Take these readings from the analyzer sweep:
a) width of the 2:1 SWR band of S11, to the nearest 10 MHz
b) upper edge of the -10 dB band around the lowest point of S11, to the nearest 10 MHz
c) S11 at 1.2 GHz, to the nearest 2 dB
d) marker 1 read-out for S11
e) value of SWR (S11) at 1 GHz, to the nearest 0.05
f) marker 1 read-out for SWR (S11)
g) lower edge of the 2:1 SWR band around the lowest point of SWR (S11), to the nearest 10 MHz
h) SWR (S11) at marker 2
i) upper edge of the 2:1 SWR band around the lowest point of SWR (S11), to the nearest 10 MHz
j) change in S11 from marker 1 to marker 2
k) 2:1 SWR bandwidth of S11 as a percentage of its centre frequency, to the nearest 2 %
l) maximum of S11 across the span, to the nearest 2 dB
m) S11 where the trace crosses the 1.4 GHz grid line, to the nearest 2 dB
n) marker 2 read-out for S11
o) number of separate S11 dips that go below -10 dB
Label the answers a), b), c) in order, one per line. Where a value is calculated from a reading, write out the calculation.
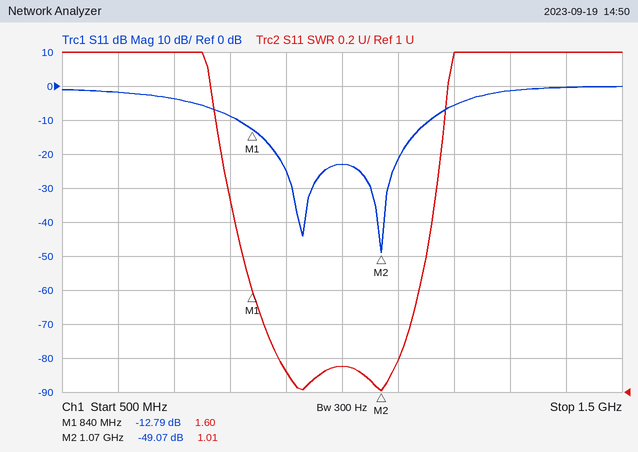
a) 1.16 GHz − 810 MHz = 350 MHz
b) 1.16 GHz
c) -6 dB
d) -12.79 dB
e) 1.15
f) 1.60
g) 810 MHz
h) 1.01
i) 1.16 GHz
j) -49.07 − (-12.79) = -36.28 dB
k) 350 MHz / 985 MHz ≈ 36 %
l) 0 dB
m) 0 dB
n) -49.07 dB
o) 2
